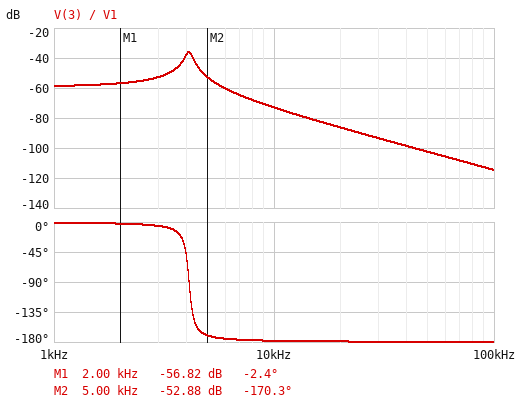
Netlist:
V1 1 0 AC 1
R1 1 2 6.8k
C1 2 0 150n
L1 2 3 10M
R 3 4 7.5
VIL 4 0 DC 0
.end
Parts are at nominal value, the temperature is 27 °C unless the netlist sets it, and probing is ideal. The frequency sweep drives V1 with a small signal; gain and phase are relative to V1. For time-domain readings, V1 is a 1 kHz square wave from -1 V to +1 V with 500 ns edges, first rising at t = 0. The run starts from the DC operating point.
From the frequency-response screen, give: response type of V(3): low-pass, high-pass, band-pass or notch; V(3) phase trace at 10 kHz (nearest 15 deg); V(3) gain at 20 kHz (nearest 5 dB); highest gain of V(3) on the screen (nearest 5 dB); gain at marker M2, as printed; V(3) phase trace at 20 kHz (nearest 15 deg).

low-pass
-180 deg
-85 dB
-35 dB
-52.88 dB
-180 deg
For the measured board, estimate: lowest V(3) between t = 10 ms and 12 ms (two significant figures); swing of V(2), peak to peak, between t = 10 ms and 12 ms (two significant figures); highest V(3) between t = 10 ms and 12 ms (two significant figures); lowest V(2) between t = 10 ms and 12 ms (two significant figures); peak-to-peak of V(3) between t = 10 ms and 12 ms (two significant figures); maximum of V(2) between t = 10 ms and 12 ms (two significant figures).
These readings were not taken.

-2.3 mV
90 mV
2.3 mV
-45 mV
4.6 mV
45 mV
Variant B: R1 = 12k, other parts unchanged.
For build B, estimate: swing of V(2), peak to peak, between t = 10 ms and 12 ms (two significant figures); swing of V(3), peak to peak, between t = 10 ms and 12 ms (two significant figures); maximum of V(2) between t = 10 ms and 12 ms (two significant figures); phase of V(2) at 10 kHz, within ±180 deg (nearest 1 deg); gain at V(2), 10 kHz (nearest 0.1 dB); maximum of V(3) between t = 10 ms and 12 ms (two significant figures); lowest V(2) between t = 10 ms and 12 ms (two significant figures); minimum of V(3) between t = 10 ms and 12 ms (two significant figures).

50 mV
2.6 mV
25 mV
-89 deg
-39.5 dB
1.3 mV
-25 mV
-1.3 mV
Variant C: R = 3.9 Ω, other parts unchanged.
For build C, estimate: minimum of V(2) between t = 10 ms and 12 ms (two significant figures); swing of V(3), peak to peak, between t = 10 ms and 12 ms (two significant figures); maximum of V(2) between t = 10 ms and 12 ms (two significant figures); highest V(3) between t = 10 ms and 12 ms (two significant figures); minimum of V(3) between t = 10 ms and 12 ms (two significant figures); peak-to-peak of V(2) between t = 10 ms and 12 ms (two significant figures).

-44 mV
2.4 mV
44 mV
1.2 mV
-1.2 mV
87 mV
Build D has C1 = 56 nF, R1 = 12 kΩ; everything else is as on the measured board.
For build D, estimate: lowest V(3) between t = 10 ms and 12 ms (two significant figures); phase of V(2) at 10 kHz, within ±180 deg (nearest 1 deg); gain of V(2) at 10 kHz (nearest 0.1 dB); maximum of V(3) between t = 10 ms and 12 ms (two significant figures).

-2.1 mV
-87 deg
-27.3 dB
2.1 mV
